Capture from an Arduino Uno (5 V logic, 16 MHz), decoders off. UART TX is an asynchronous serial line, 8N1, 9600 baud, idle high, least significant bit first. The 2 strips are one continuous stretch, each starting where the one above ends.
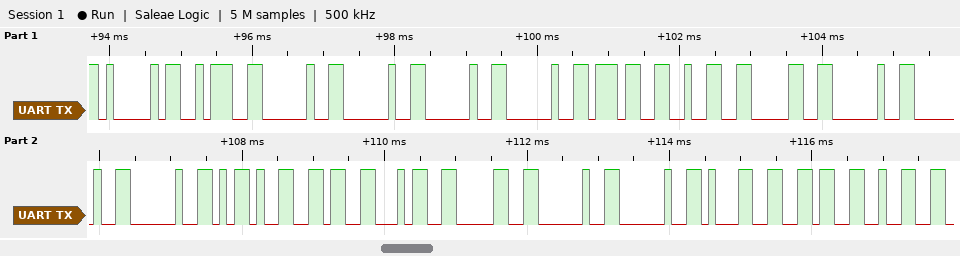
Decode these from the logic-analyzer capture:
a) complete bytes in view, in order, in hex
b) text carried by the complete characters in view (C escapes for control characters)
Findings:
41 3A 20 20 20 20 37 32 30 20 20 20 2D 36 34 30 20 20 31 36 32
"A:    720   -640  162"
